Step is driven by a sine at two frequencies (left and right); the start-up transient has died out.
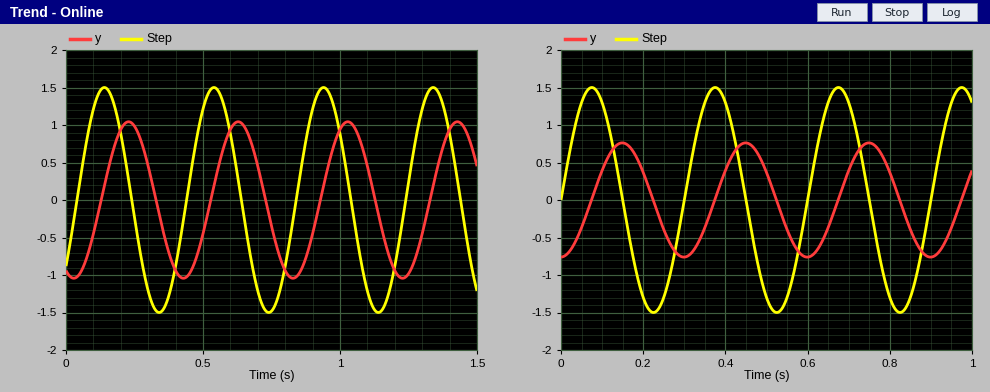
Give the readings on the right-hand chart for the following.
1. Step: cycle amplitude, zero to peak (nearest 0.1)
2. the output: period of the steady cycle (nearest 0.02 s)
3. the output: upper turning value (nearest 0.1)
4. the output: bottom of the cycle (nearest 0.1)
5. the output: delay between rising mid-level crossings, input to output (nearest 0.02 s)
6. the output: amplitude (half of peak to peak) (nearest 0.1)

1.5
0.30 s
0.8
-0.8
0.08 s
0.8
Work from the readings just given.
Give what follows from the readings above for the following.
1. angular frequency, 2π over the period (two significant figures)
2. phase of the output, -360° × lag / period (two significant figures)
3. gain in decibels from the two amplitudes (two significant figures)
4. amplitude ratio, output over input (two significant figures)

21 rad/s
-96°
-5.5 dB
0.53
